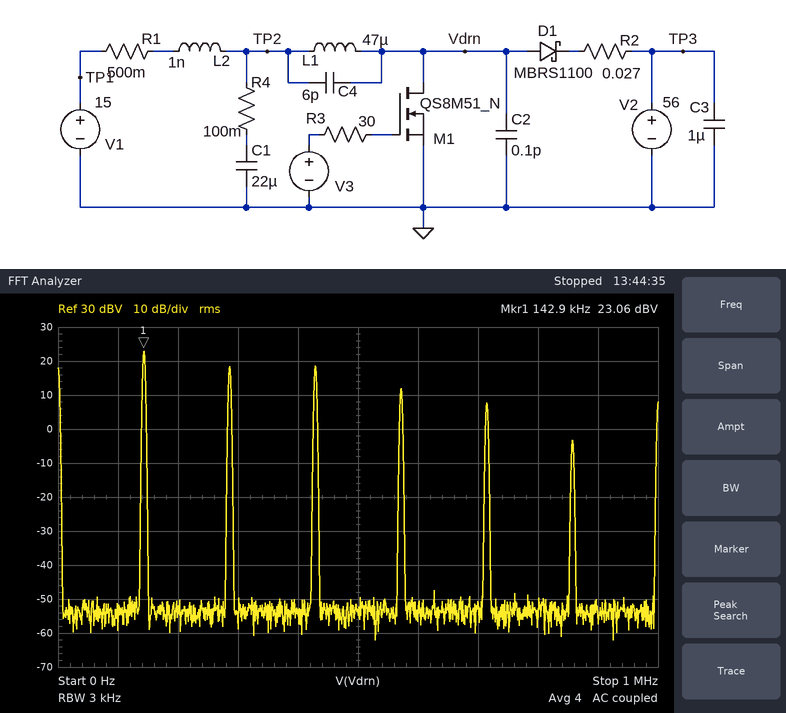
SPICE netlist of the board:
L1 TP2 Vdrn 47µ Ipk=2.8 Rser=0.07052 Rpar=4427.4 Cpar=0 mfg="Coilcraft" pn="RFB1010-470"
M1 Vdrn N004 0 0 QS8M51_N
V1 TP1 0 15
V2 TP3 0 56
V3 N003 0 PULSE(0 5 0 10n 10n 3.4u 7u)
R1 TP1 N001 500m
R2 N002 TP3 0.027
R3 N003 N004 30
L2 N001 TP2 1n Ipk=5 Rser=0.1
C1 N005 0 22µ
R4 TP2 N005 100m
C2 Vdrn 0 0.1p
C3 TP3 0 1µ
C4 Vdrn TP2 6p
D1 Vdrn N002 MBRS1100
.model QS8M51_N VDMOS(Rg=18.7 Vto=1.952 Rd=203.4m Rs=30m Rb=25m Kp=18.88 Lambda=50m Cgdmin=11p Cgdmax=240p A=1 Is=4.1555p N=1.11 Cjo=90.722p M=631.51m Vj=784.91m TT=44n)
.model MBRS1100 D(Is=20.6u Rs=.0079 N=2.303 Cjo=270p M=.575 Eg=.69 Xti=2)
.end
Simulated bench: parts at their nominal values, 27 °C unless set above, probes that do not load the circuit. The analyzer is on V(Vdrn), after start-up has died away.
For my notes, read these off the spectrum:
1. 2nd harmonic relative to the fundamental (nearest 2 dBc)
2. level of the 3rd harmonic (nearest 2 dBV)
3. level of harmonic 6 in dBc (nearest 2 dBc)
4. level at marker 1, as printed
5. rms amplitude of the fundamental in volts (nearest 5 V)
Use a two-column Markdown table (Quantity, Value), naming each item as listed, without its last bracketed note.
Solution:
| Quantity | Value |
|---|---|
| 2nd harmonic relative to the fundamental | -4 dBc |
| level of the 3rd harmonic | 18 dBV |
| level of harmonic 6 in dBc | -26 dBc |
| level at marker 1, as printed | 23.06 dBV |
| rms amplitude of the fundamental in volts | 15 V |
